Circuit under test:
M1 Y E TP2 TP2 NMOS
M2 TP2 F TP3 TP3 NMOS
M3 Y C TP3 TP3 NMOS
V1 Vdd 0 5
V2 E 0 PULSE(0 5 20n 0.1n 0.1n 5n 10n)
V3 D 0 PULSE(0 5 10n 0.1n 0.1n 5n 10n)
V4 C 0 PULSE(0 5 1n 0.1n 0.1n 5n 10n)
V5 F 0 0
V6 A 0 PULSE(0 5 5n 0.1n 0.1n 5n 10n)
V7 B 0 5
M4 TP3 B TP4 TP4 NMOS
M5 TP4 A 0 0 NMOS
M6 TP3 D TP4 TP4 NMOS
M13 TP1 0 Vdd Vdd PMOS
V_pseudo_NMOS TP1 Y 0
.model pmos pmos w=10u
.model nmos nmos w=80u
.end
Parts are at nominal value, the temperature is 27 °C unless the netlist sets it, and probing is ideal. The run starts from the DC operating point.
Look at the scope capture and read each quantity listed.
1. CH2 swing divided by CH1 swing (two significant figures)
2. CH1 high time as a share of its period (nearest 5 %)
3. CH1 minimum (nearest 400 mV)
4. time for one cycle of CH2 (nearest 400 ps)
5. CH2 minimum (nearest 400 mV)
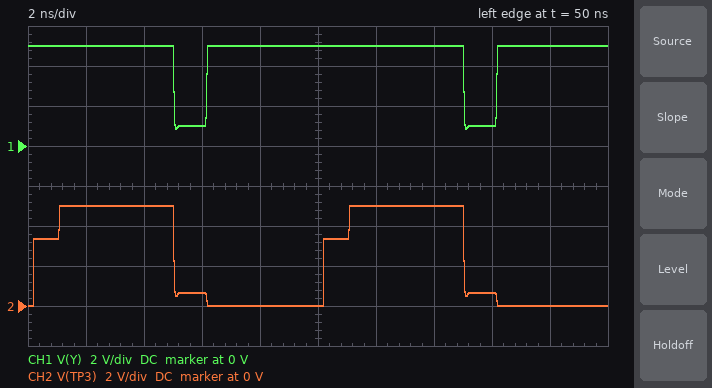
1.2
90 %
800 mV
10.0 ns
0 V
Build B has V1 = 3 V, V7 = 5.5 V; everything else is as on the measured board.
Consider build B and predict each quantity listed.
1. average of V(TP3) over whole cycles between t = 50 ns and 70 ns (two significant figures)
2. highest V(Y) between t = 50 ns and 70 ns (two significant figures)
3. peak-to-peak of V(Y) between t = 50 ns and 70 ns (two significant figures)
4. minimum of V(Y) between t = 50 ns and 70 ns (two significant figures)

1.4 V
3.0 V
2.7 V
280 mV
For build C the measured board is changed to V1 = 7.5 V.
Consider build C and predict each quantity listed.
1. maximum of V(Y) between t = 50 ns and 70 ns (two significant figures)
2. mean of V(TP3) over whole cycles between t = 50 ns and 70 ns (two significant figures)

7.5 V
2.5 V
